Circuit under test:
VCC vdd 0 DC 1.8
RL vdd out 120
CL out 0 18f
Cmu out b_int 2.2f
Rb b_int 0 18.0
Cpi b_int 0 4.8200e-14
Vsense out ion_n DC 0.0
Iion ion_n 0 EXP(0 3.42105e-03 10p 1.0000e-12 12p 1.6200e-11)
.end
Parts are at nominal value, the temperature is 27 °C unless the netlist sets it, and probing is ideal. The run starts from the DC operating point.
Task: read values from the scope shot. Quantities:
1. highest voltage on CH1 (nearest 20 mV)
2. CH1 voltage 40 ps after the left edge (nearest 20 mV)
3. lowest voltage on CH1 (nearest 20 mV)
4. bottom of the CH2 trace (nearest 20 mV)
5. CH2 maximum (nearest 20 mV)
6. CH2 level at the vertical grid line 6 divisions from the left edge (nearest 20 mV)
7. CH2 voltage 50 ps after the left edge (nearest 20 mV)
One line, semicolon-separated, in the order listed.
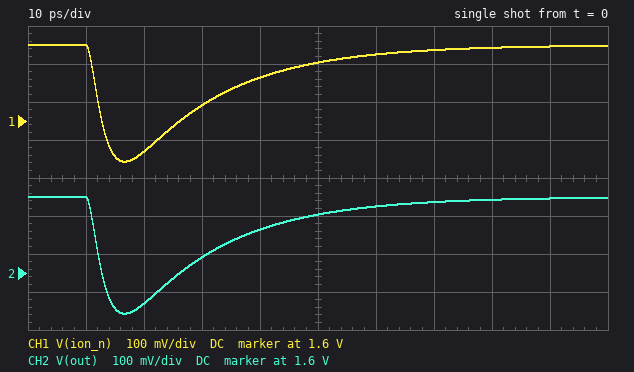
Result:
1.80 V; 1.72 V; 1.50 V; 1.50 V; 1.80 V; 1.78 V; 1.76 V
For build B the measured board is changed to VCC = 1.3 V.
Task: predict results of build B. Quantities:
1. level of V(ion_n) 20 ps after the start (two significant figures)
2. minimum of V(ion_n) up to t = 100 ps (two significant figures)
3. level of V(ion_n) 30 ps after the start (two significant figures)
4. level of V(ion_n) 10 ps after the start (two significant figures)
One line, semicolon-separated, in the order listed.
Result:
1.0 V; 990 mV; 1.1 V; 1.3 V
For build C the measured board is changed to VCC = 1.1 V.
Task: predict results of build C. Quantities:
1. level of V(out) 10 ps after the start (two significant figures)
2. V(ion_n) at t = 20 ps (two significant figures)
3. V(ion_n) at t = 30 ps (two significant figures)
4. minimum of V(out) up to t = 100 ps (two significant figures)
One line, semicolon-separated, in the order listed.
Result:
1.1 V; 820 mV; 940 mV; 790 mV
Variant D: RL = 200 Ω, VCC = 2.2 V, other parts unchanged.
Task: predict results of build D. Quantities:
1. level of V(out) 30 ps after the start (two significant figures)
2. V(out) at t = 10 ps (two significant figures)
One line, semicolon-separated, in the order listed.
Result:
1.9 V; 2.2 V
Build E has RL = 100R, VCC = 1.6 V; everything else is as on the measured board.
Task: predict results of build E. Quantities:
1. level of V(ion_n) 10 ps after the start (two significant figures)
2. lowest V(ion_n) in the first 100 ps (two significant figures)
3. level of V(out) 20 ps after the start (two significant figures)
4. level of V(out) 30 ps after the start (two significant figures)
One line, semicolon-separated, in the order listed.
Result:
1.6 V; 1.3 V; 1.4 V; 1.5 V
